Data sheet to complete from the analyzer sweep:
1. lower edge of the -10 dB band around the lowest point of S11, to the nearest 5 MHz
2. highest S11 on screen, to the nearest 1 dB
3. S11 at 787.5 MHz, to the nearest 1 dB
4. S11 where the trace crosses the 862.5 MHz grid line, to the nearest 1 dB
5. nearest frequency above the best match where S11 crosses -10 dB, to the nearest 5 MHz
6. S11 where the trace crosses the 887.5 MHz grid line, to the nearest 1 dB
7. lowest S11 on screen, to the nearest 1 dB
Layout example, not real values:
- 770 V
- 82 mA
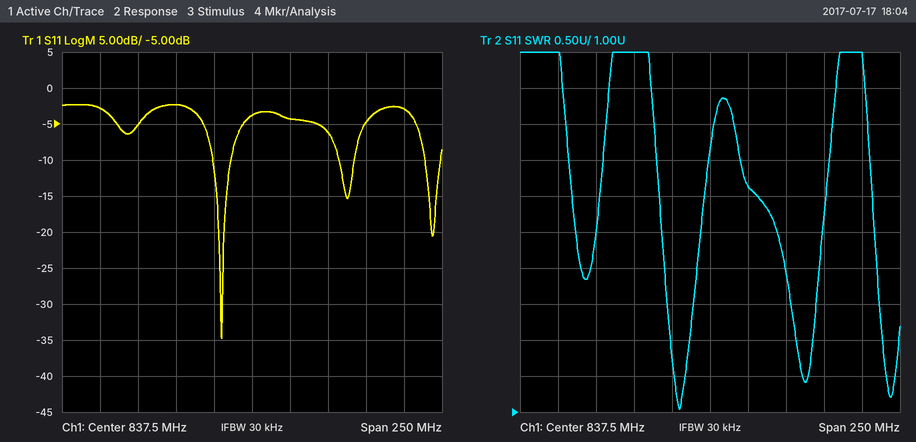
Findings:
- 810 MHz
- -2 dB
- -2 dB
- -4 dB
- 825 MHz
- -6 dB
- -35 dB
